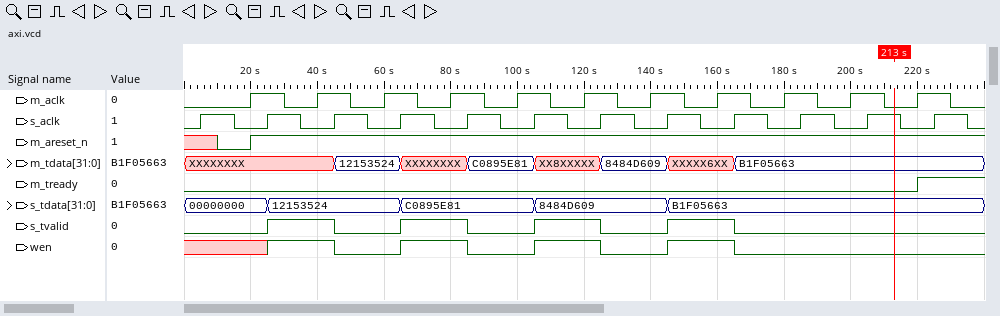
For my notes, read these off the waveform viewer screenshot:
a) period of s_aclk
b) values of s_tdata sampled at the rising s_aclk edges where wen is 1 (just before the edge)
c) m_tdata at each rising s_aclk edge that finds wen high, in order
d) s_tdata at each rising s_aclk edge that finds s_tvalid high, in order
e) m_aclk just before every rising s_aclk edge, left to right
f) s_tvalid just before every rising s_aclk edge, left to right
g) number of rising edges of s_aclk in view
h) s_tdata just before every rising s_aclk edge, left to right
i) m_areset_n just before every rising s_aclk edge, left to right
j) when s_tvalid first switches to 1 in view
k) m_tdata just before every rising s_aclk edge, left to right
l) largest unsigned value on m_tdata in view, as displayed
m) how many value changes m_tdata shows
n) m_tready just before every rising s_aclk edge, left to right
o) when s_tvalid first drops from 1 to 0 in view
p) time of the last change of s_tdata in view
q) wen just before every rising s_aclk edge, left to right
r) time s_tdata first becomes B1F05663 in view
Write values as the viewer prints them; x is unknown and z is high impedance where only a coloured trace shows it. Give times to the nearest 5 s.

20 s
12153524, C0895E81, 8484D609, B1F05663
XXXXXXXX, XXXXXXXX, XX8XXXXX, XXXXX6XX
12153524, C0895E81, 8484D609, B1F05663
0 1 1 1 1 1 1 1 1 1 1 1
0 0 1 0 1 0 1 0 1 0 0 0
12
00000000, 00000000, 12153524, 12153524, C0895E81, C0895E81, 8484D609, 8484D609, B1F05663, B1F05663, B1F05663, B1F05663
x 1 1 1 1 1 1 1 1 1 1 1
25 s
XXXXXXXX, XXXXXXXX, XXXXXXXX, 12153524, XXXXXXXX, C0895E81, XX8XXXXX, 8484D609, XXXXX6XX, B1F05663, B1F05663, B1F05663
C0895E81
7
0 0 0 0 0 0 0 0 0 0 0 1
45 s
145 s
x x 1 0 1 0 1 0 1 0 0 0
145 s
